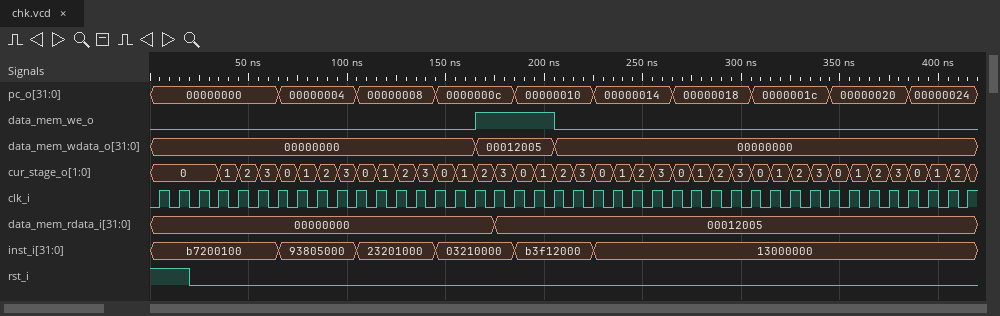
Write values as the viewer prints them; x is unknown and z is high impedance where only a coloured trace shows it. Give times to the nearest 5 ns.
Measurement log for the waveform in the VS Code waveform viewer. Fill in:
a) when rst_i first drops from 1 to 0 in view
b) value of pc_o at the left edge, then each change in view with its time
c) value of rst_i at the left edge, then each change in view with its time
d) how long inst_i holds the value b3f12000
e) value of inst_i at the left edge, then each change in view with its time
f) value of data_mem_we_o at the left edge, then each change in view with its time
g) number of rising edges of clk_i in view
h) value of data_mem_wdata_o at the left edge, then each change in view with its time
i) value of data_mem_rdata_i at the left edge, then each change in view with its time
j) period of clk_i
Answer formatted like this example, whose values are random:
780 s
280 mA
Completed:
20 ns
00000000, 00000004 at 65 ns, 00000008 at 105 ns, 0000000c at 145 ns, 00000010 at 185 ns, 00000014 at 225 ns, 00000018 at 265 ns, 0000001c at 305 ns, 00000020 at 345 ns, 00000024 at 385 ns
1, 0 at 20 ns
40 ns
b7200100, 93805000 at 65 ns, 23201000 at 105 ns, 03210000 at 145 ns, b3f12000 at 185 ns, 13000000 at 225 ns
0, 1 at 165 ns, 0 at 205 ns
42
00000000, 00012005 at 165 ns, 00000000 at 205 ns
00000000, 00012005 at 175 ns
10 ns
